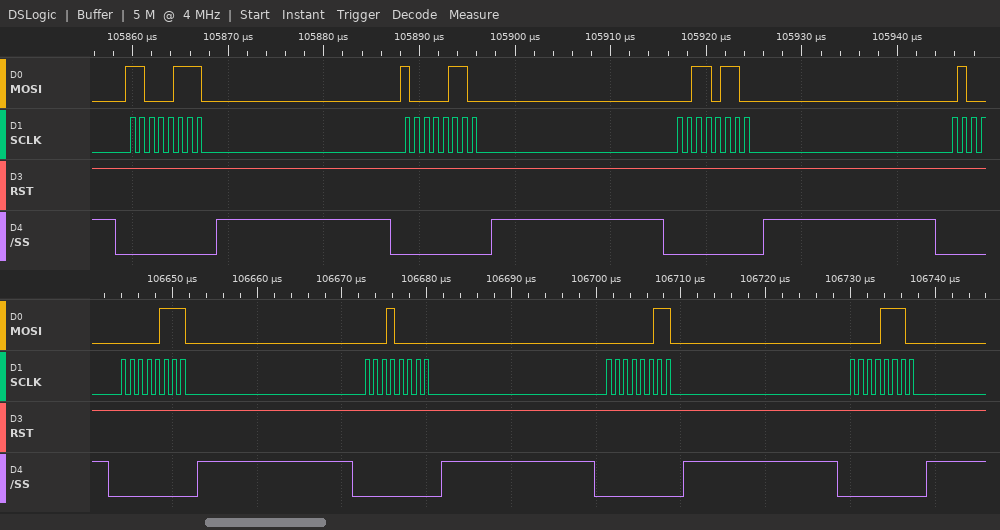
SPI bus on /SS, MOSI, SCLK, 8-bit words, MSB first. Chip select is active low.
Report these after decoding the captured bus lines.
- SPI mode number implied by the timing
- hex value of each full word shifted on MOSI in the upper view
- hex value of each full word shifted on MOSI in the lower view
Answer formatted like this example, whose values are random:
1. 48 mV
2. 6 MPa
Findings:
1. 0
2. C7, 86, 36
3. 07, 10, 03, 0E
